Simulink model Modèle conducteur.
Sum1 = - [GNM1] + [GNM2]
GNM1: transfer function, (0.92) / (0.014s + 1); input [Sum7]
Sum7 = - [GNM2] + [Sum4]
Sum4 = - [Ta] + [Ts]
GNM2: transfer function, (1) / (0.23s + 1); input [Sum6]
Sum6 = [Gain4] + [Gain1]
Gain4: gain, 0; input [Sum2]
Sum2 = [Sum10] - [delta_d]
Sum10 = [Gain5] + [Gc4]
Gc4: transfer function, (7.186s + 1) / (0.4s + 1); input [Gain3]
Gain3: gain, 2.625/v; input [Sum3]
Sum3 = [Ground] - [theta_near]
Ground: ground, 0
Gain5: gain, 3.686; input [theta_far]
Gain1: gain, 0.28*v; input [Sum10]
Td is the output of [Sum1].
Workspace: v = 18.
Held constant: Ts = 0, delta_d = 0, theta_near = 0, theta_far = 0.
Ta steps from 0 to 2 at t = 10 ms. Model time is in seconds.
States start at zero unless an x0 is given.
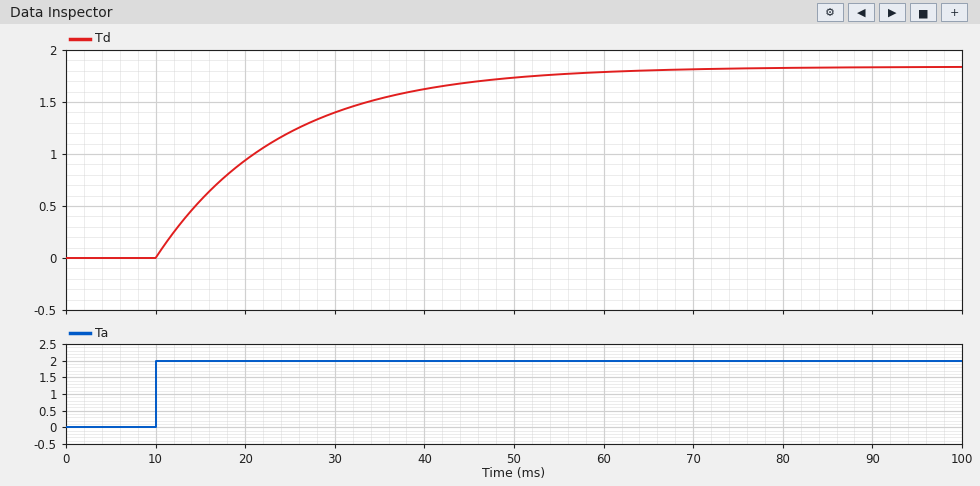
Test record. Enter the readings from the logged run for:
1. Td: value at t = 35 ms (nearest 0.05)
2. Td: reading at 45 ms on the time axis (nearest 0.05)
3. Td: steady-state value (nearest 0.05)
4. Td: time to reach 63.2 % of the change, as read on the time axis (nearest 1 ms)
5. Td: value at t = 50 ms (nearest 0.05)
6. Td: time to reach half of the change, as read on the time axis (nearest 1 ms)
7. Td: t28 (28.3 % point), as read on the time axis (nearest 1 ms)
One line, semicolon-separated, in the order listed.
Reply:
1.55; 1.70; 1.85; 24 ms; 1.75; 20 ms; 15 ms
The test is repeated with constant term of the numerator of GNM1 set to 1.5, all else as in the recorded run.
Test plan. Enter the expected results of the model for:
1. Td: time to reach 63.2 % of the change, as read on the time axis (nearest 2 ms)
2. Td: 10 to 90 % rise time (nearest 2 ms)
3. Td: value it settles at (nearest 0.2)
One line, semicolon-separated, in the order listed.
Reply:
24 ms; 30 ms; 3.0
